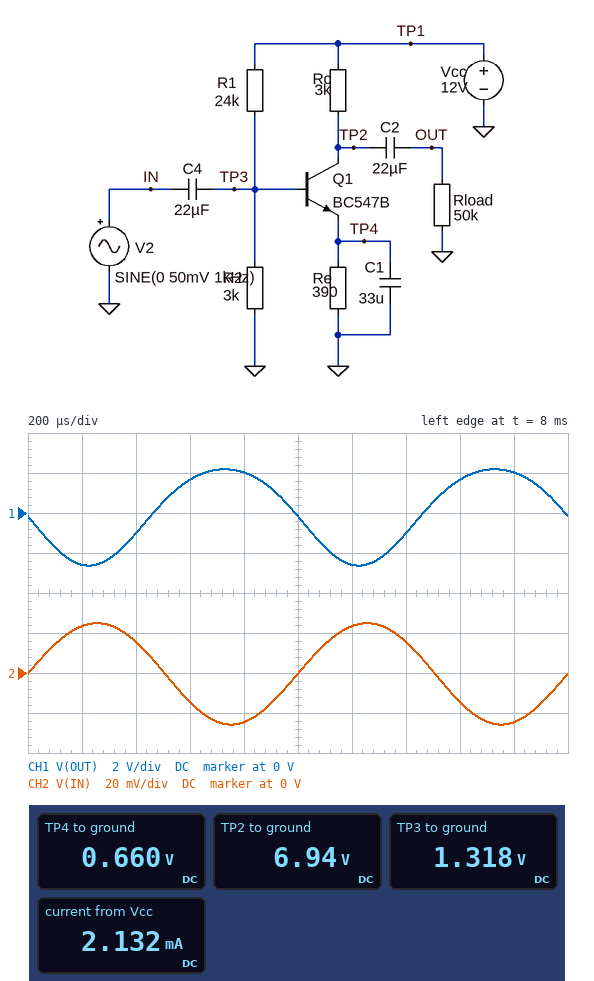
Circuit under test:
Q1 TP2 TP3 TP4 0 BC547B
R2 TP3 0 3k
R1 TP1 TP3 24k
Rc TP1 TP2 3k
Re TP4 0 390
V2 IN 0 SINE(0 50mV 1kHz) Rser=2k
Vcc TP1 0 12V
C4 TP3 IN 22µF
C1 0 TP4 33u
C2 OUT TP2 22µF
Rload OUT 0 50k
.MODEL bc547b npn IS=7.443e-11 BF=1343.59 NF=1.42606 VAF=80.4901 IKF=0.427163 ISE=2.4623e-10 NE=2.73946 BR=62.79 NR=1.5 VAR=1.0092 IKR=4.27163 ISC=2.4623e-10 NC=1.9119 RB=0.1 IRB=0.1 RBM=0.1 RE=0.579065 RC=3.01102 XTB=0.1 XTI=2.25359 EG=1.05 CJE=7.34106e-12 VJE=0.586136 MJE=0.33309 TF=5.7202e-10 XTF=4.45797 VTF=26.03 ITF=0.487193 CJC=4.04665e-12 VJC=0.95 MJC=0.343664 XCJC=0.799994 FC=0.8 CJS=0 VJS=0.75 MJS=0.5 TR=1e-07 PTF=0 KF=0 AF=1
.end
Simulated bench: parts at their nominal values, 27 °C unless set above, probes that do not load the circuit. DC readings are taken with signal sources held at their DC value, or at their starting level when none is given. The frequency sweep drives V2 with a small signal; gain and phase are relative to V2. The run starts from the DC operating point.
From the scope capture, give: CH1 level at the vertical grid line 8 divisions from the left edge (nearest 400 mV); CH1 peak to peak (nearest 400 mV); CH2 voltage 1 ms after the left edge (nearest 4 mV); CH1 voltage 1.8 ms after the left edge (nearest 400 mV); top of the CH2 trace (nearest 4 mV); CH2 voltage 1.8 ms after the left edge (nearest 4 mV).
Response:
1.6 V
4.8 V
0 V
2.0 V
24 mV
-24 mV
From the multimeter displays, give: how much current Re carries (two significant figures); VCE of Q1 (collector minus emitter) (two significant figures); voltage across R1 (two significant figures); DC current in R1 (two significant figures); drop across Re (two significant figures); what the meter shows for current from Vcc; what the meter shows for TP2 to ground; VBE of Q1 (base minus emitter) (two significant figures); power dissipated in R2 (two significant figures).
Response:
1.7 mA
6.3 V
11 V
450 µA
660 mV
2.132 mA
6.94 V
660 mV
580 µW
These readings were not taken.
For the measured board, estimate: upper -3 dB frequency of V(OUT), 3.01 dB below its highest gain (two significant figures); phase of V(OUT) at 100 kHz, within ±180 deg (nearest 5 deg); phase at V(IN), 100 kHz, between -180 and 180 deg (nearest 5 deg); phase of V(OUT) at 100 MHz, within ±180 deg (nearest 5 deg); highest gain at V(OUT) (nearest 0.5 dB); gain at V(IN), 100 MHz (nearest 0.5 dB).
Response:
620 kHz
170 deg
-10 deg
60 deg
34.0 dB
-40.5 dB
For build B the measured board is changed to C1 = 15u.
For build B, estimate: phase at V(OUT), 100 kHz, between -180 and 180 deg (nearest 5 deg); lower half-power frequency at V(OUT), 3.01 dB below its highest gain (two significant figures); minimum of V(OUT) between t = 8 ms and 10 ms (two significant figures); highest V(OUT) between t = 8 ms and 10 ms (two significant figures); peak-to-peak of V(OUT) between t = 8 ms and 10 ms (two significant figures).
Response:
170 deg
360 Hz
-2.5 V
2.1 V
4.6 V
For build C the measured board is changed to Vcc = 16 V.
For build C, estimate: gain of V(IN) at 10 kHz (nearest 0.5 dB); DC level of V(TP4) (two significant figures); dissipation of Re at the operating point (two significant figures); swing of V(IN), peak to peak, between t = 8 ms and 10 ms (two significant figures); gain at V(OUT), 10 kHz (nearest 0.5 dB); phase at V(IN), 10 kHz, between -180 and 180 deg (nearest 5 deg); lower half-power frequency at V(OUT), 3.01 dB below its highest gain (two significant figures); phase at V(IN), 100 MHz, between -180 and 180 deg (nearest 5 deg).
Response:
-6.5 dB
1.1 V
3.0 mW
48 mV
37.0 dB
0 deg
220 Hz
-40 deg
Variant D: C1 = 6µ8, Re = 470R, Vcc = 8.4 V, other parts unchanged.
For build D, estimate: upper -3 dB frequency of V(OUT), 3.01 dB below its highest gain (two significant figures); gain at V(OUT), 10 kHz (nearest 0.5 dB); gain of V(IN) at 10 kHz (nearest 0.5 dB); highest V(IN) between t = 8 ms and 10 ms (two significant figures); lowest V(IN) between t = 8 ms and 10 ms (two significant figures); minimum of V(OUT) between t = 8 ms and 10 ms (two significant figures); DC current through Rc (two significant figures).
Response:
1.2 MHz
27.5 dB
-5.5 dB
27 mV
-27 mV
-1.2 V
650 µA
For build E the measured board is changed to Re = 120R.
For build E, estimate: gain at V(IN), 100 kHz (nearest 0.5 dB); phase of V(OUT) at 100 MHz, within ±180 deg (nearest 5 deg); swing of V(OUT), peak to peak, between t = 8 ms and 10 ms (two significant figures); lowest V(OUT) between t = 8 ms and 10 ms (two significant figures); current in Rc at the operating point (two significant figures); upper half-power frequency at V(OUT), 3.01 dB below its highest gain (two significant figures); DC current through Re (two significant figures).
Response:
-34.5 dB
-15 deg
51 mV
-19 mV
3.8 mA
180 kHz
3.9 mA
